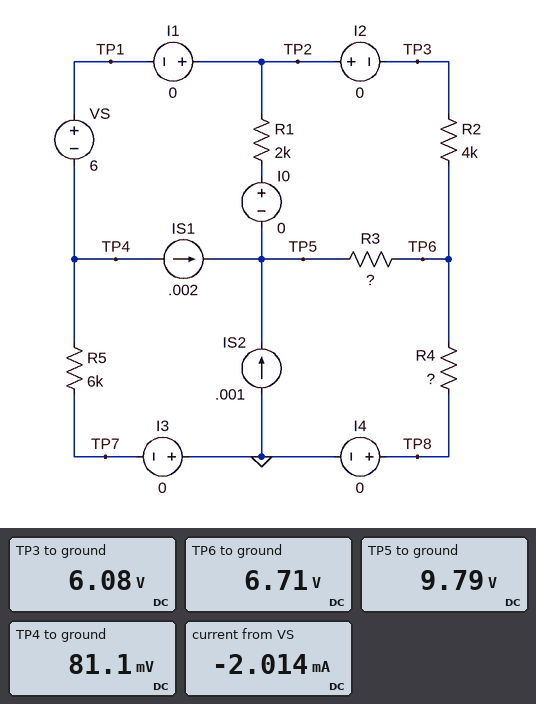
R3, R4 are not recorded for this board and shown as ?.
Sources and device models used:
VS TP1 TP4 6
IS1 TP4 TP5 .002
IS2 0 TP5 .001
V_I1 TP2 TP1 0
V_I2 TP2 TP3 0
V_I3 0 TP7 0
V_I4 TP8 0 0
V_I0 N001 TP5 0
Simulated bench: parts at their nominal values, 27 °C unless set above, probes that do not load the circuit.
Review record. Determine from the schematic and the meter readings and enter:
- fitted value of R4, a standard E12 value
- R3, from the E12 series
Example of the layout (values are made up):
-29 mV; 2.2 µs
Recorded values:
6.8 kΩ; 2.7 kΩ
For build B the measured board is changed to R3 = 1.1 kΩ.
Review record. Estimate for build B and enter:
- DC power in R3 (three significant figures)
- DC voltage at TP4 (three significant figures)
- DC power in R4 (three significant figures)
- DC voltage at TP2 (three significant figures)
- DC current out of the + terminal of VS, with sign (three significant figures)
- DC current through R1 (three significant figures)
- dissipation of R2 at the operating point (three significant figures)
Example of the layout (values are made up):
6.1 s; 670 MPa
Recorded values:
2.28 mW; -344 mV; 7.60 mW; 5.66 V; -1.94 mA; 1.56 mA; 588 µW
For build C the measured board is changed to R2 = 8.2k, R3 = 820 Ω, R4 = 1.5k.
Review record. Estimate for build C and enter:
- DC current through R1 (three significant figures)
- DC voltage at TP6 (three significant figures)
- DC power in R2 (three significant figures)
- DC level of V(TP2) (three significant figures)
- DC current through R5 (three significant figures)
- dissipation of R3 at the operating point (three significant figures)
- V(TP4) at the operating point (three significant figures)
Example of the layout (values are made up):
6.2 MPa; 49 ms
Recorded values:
1.18 mA; 2.57 V; 91.3 µW; 1.71 V; 715 µA; 2.72 mW; -4.29 V
